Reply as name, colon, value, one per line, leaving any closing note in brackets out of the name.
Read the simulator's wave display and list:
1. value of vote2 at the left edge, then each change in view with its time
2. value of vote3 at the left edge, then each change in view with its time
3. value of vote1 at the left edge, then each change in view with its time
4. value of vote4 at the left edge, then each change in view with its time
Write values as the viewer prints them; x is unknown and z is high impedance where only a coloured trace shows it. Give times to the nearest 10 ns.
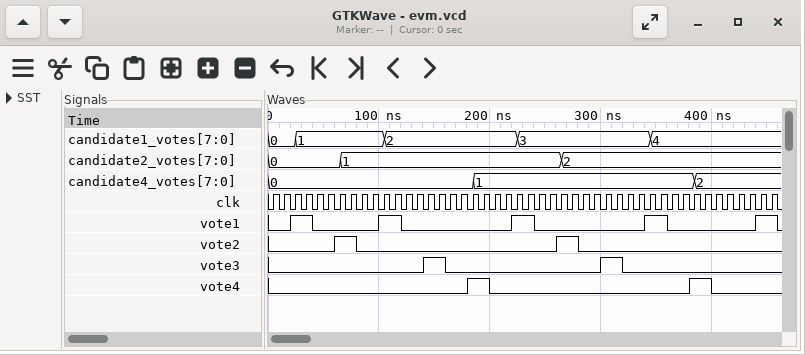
value of vote2 at the left edge, then each change in view with its time: 0, 1 at 60 ns, 0 at 80 ns, 1 at 260 ns, 0 at 280 ns
value of vote3 at the left edge, then each change in view with its time: 0, 1 at 140 ns, 0 at 160 ns, 1 at 300 ns, 0 at 320 ns
value of vote1 at the left edge, then each change in view with its time: 0, 1 at 20 ns, 0 at 40 ns, 1 at 100 ns, 0 at 120 ns, 1 at 220 ns, 0 at 240 ns, 1 at 340 ns, 0 at 360 ns, 1 at 440 ns, 0 at 460 ns
value of vote4 at the left edge, then each change in view with its time: 0, 1 at 180 ns, 0 at 200 ns, 1 at 380 ns, 0 at 400 ns
